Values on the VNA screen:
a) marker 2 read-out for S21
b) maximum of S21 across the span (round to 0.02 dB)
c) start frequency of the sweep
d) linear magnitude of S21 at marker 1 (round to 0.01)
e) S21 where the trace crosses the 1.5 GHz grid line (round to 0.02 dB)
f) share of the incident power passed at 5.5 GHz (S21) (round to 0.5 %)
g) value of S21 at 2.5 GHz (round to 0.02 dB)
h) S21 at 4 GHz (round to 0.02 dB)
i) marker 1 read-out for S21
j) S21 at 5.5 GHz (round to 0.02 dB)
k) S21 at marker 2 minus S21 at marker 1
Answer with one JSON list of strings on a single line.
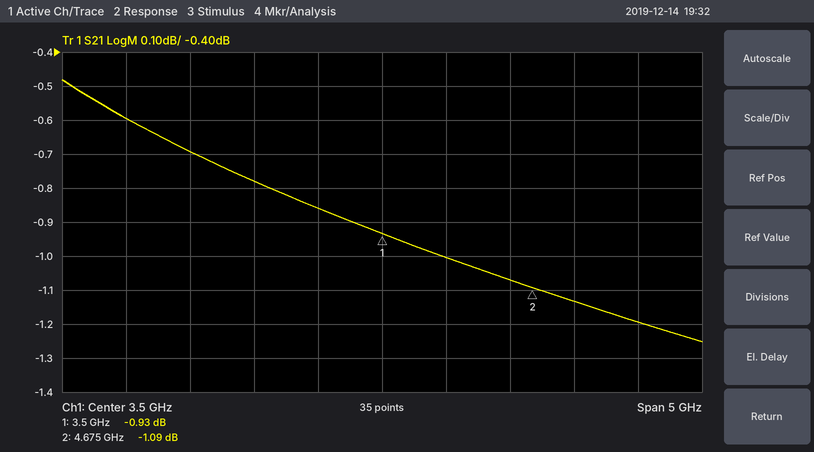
["-1.09 dB", "-0.48 dB", "1 GHz", "0.90", "-0.60 dB", "76.0 %", "-0.78 dB", "-1.00 dB", "-0.93 dB", "-1.20 dB", "-0.16 dB"]
